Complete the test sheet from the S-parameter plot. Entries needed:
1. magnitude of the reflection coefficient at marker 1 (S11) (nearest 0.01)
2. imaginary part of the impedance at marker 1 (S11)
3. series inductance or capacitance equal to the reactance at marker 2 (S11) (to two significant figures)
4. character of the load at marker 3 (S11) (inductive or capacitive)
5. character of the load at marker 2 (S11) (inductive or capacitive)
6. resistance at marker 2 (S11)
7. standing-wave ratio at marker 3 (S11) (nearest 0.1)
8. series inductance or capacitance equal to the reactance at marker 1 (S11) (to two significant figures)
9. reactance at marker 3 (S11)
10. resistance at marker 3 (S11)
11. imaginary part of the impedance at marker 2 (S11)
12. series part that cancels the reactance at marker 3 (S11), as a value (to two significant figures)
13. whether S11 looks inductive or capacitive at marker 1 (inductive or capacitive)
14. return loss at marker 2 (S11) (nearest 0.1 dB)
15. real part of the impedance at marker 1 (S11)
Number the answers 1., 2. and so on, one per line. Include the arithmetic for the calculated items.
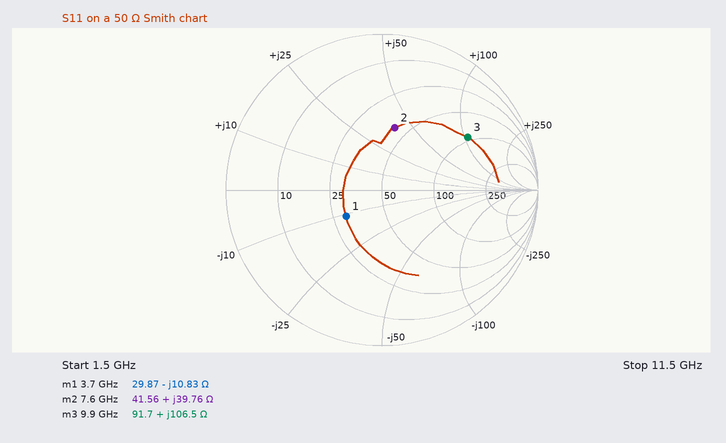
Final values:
1. 0.28
2. -10.83 Ω
3. L = 39.76 Ω/(2π × 7.6 GHz) ≈ 833 pH, so 830 pH to two significant figures
4. inductive
5. inductive
6. 41.56 Ω
7. 4.6
8. C = 1/(2π × 3.7 GHz × 10.83 Ω) ≈ 4.0 pF
9. +106.5 Ω
10. 91.7 Ω
11. +39.76 Ω
12. C = 1/(2π × 9.9 GHz × 106.5 Ω) ≈ 151 fF, so 150 fF to two significant figures
13. capacitive
14. 7.8 dB
15. 29.87 Ω
